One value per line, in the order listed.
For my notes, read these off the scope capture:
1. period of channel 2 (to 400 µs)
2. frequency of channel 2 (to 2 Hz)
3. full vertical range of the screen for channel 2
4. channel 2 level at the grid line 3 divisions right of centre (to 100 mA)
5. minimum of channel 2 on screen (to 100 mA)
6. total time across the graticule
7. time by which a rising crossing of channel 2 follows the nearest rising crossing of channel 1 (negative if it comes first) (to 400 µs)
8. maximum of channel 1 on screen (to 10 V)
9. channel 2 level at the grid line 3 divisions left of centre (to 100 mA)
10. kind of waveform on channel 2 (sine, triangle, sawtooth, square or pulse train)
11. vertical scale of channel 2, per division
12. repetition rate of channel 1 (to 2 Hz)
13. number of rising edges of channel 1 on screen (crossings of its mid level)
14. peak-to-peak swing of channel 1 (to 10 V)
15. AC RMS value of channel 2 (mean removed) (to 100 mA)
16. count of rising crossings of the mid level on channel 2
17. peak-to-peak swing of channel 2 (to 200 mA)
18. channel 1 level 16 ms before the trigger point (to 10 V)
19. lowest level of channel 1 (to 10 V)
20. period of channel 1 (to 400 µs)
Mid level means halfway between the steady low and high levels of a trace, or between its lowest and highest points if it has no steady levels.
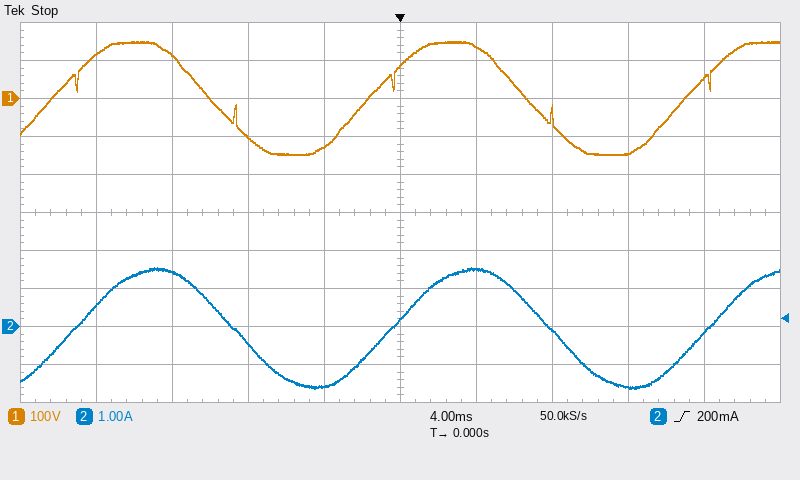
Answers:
16.8 ms
60 Hz
10 A
-1.6 A
-1.6 A
40 ms
+1.2 ms
150 V
1.4 A
sine
1 A
60 Hz
3
300 V
1.1 A
3
3.2 A
120 V
-150 V
16.8 ms
